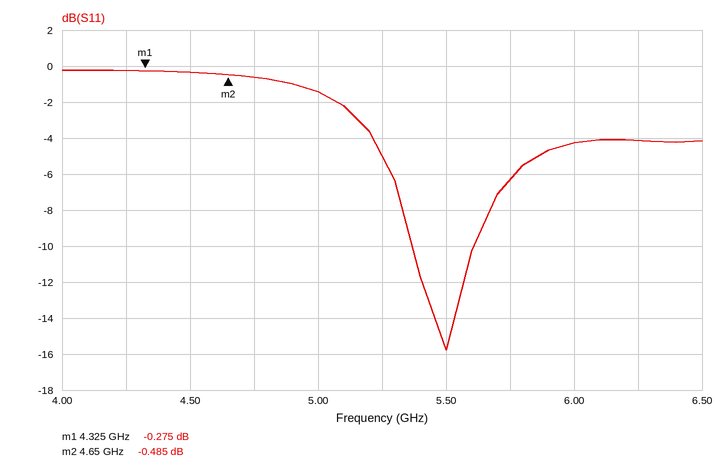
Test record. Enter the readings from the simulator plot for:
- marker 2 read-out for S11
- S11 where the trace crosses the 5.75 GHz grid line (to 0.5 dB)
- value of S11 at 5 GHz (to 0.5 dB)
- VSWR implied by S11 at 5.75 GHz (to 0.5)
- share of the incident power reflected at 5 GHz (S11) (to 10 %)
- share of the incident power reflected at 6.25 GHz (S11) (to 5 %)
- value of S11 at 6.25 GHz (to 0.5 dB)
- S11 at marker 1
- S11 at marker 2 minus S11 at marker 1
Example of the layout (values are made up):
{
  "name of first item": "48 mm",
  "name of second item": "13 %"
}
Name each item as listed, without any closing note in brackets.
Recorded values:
{
  "marker 2 read-out for S11": "-0.485 dB",
  "S11 where the trace crosses the 5.75 GHz grid line": "-6.5 dB",
  "value of S11 at 5 GHz": "-1.5 dB",
  "VSWR implied by S11 at 5.75 GHz": "3.0",
  "share of the incident power reflected at 5 GHz (S11)": "70 %",
  "share of the incident power reflected at 6.25 GHz (S11)": "40 %",
  "value of S11 at 6.25 GHz": "-4.0 dB",
  "S11 at marker 1": "-0.275 dB",
  "S11 at marker 2 minus S11 at marker 1": "-0.210 dB"
}
